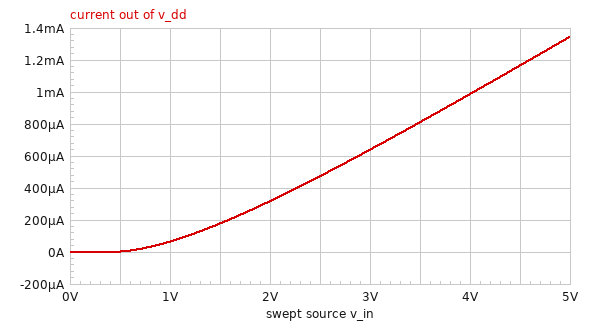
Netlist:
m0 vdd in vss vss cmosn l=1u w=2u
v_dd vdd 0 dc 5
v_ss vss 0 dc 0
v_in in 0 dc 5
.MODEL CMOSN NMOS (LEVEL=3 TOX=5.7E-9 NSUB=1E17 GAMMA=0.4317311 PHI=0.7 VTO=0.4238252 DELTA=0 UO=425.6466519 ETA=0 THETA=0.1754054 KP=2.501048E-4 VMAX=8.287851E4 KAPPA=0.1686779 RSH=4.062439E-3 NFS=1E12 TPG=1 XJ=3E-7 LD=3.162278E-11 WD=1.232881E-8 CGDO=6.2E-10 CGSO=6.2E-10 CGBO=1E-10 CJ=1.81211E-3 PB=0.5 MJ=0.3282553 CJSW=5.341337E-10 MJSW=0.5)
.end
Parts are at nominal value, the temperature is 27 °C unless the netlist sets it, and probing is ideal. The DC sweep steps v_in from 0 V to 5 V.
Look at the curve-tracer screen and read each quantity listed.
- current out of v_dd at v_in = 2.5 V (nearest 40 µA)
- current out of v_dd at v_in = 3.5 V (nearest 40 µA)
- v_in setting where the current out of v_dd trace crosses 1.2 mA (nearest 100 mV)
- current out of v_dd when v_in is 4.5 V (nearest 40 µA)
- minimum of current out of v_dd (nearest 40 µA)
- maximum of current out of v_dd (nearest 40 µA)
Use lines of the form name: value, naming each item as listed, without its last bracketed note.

current out of v_dd at v_in = 2.5 V: 480 µA
current out of v_dd at v_in = 3.5 V: 800 µA
v_in setting where the current out of v_dd trace crosses 1.2 mA: 4.6 V
current out of v_dd when v_in is 4.5 V: 1.16 mA
minimum of current out of v_dd: 0 A
maximum of current out of v_dd: 1.36 mA
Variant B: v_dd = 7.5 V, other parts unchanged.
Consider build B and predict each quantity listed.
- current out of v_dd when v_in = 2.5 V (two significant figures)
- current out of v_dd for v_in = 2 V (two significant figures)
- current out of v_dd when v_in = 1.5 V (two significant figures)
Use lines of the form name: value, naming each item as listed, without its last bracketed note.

current out of v_dd when v_in = 2.5 V: 490 µA
current out of v_dd for v_in = 2 V: 330 µA
current out of v_dd when v_in = 1.5 V: 180 µA
